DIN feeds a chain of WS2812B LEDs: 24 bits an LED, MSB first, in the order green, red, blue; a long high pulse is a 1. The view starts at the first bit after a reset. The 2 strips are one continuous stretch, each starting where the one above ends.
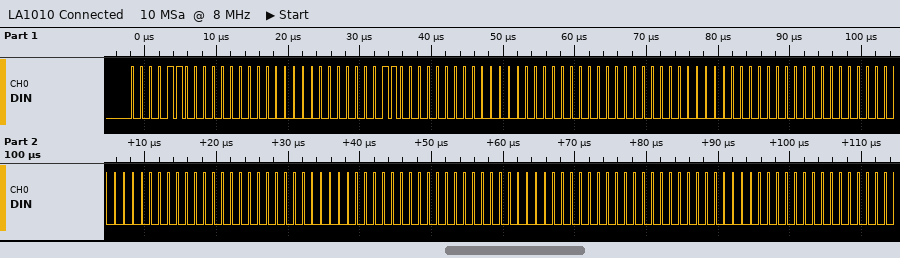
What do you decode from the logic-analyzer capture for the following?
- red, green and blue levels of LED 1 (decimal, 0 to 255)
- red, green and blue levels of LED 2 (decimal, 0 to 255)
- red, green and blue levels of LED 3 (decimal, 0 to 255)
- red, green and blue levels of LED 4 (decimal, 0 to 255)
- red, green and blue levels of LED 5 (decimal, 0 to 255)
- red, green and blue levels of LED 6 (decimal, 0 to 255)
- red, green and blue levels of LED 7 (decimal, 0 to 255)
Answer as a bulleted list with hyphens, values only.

- 0, 12, 0
- 0, 12, 0
- 0, 0, 0
- 0, 0, 0
- 0, 0, 0
- 0, 0, 0
- 0, 0, 0
